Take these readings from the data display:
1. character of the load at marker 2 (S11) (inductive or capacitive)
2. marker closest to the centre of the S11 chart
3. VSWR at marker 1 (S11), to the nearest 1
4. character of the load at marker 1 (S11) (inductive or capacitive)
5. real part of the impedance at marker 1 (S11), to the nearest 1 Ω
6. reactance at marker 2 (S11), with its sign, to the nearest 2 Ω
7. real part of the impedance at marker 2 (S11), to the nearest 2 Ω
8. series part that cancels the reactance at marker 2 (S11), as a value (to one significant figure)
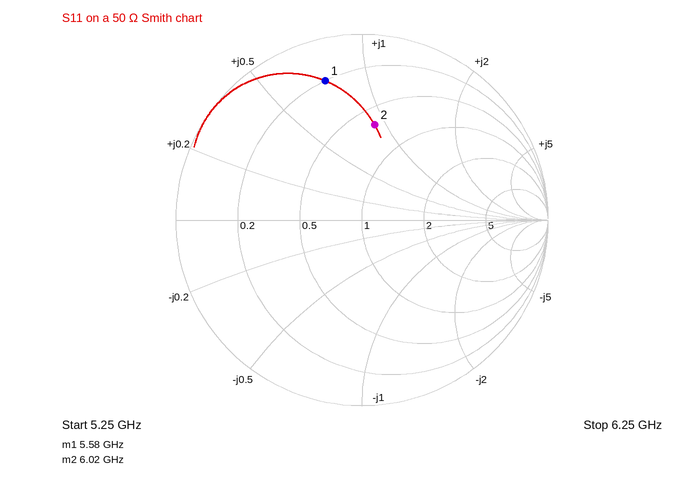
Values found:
inductive
marker 2
8
inductive
10 Ω
+46 Ω
32 Ω
600 fF
